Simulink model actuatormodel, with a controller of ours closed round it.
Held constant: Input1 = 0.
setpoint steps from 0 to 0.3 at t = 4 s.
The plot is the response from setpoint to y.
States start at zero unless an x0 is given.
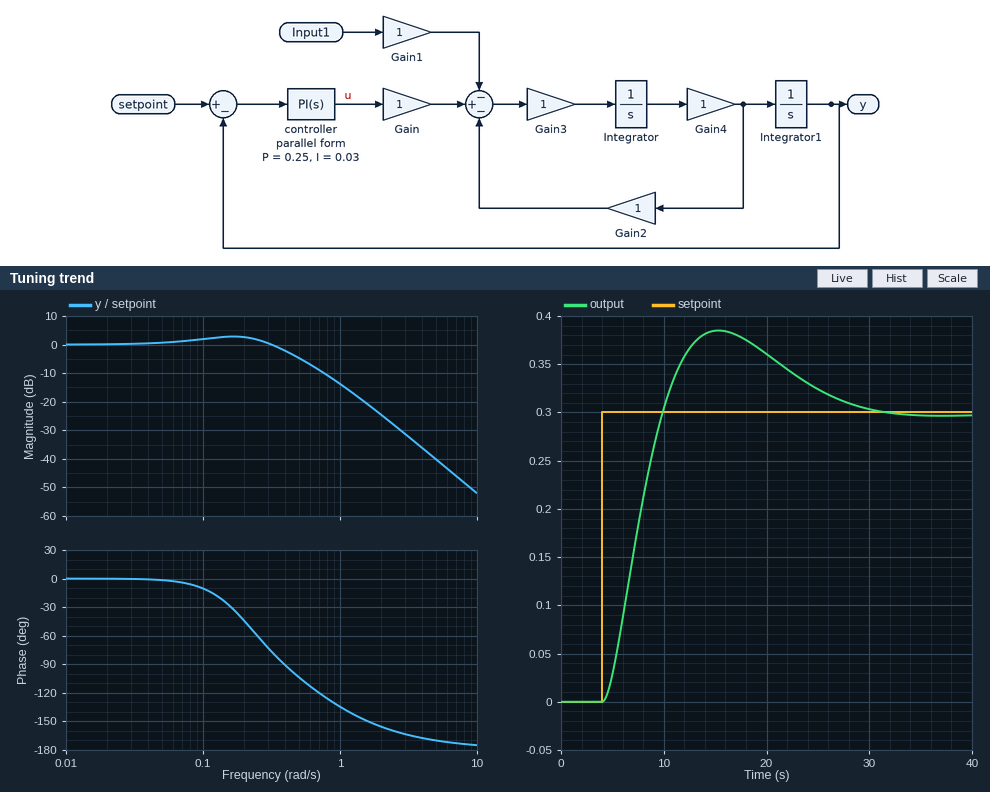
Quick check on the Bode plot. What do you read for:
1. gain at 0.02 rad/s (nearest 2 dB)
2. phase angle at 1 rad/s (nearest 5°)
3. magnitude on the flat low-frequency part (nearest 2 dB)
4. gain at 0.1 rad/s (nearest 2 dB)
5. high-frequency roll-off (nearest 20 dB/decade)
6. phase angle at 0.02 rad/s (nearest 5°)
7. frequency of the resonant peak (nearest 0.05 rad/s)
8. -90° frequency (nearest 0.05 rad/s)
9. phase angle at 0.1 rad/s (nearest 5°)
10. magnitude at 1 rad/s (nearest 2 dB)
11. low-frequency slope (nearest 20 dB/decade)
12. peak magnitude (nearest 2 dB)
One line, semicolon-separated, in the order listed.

0 dB; -135°; 0 dB; 2 dB; -40 dB/decade; 0°; 0.15 rad/s; 0.40 rad/s; -10°; -14 dB; 0 dB/decade; 2 dB
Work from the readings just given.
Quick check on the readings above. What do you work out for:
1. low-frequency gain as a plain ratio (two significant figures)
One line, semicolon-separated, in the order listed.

1.0
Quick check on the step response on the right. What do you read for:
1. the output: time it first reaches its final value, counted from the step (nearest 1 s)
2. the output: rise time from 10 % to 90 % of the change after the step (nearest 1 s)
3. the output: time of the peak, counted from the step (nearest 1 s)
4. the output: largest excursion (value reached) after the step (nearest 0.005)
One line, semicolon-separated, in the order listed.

6 s; 4 s; 11 s; 0.385
